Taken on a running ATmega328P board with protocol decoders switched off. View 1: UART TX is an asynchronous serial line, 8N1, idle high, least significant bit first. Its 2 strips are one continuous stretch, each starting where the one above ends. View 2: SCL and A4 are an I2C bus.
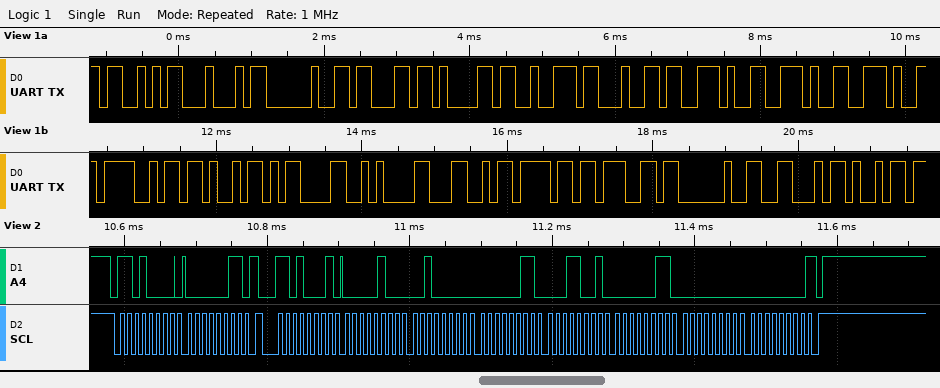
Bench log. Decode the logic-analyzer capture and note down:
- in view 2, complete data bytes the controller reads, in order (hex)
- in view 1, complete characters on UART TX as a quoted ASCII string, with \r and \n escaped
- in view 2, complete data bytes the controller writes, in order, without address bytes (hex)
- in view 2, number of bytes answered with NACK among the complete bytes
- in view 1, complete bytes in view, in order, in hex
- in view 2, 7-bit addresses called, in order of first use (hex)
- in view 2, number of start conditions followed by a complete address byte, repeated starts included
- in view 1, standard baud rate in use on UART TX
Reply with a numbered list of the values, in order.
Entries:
1. 04 20 03 19 03 00 00
2. "SD card...OK\r\nLog Fi"
3. 03
4. 1
5. 53 44 20 63 61 72 64 2E 2E 2E 4F 4B 0D 0A 4C 6F 67 20 46 69
6. 0x68
7. 2
8. 9600 baud
